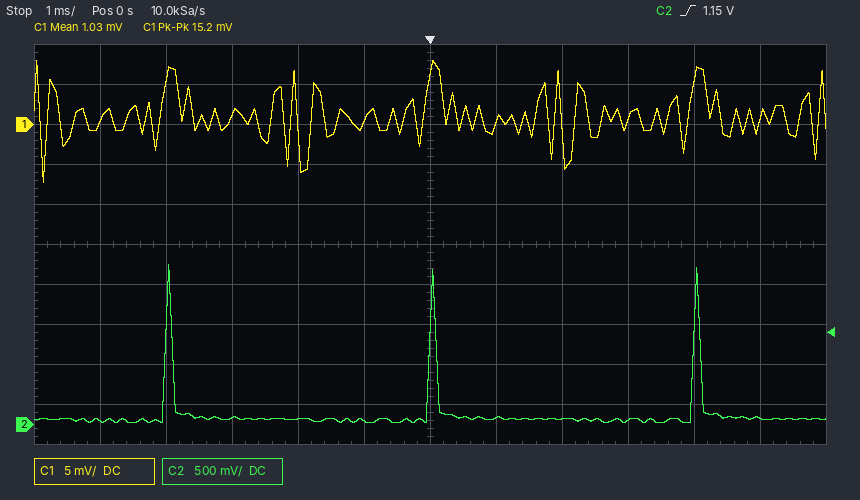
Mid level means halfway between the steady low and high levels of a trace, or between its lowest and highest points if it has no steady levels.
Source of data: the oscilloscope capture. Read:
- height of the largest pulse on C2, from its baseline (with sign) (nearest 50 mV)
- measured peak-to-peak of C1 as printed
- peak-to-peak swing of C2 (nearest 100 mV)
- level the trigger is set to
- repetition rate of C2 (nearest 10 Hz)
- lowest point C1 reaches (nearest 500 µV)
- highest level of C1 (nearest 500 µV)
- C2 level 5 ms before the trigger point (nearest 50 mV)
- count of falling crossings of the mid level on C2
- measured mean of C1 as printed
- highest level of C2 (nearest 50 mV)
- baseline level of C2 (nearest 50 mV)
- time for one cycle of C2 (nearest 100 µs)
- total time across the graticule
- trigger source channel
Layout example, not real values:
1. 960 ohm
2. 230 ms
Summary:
1. +1.95 V
2. 15.2 mV
3. 2.00 V
4. 1.15 V
5. 250 Hz
6. -7.0 mV
7. 8.0 mV
8. 50 mV
9. 3
10. 1.03 mV
11. 2.00 V
12. 50 mV
13. 4.0 ms
14. 12 ms
15. C2
